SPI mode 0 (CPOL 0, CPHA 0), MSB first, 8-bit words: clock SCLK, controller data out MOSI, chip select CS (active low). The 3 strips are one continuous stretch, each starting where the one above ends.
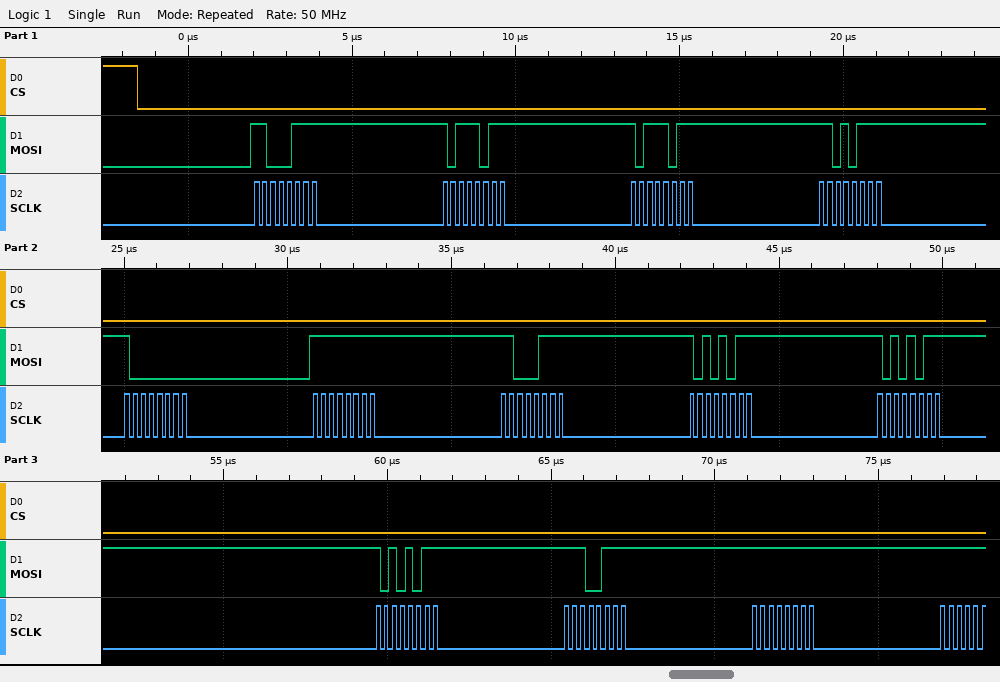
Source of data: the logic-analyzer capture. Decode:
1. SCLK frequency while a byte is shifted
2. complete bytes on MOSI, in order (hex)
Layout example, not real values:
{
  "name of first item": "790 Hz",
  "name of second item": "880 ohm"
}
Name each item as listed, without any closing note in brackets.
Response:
{
  "SCLK frequency while a byte is shifted": "4 MHz",
  "complete bytes on MOSI, in order": "C7 BB BB D7 80 FF C7 AB AB AB E7 FF"
}
